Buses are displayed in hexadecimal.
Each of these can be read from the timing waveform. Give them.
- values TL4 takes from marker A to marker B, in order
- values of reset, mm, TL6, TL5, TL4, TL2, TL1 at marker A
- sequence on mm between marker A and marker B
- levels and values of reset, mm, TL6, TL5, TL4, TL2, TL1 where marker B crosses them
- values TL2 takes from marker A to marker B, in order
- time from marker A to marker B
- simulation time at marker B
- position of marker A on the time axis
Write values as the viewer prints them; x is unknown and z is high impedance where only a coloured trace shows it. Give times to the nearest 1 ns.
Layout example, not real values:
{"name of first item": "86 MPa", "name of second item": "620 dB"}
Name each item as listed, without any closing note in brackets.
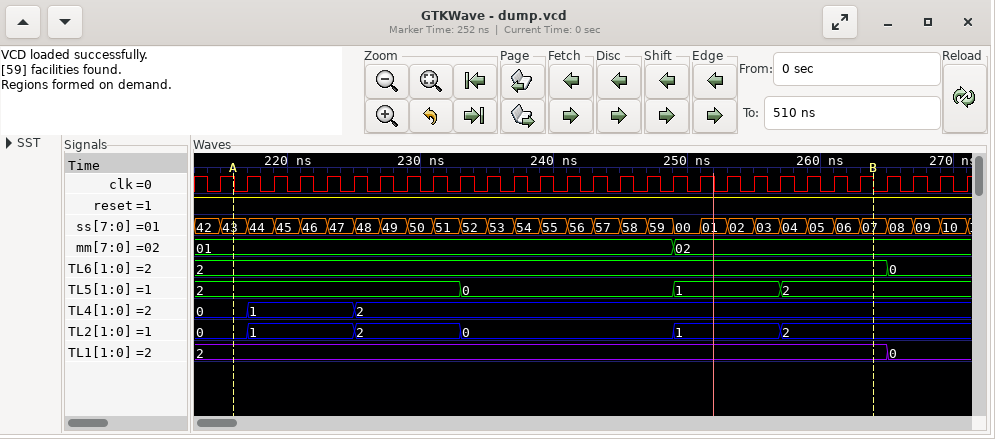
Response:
{"values TL4 takes from marker A to marker B, in order": "0, 1, 2", "values of reset, mm, TL6, TL5, TL4, TL2, TL1 at marker A": "reset=1, mm=01, TL6=2, TL5=2, TL4=0, TL2=0, TL1=2", "sequence on mm between marker A and marker B": "01, 02", "levels and values of reset, mm, TL6, TL5, TL4, TL2, TL1 where marker B crosses them": "reset=1, mm=02, TL6=2, TL5=2, TL4=2, TL2=2, TL1=2", "values TL2 takes from marker A to marker B, in order": "0, 1, 2, 0, 1, 2", "time from marker A to marker B": "48 ns", "simulation time at marker B": "264 ns", "position of marker A on the time axis": "216 ns"}
